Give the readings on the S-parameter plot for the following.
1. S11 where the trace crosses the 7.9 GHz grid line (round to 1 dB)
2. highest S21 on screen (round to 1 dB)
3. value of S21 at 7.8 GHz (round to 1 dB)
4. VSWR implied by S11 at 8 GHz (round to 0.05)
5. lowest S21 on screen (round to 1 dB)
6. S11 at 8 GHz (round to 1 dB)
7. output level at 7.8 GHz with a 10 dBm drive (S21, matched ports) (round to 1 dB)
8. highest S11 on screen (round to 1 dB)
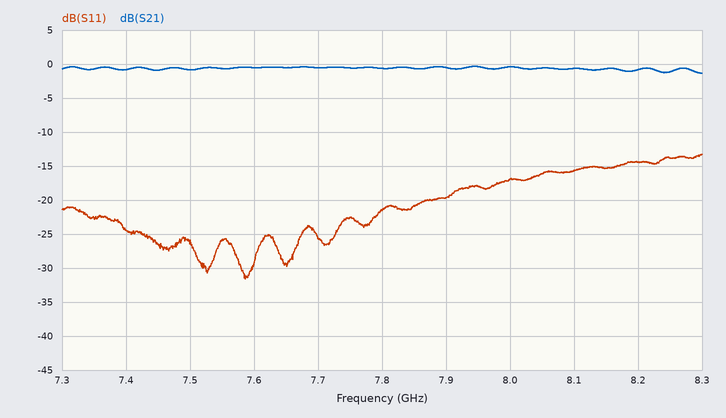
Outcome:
-20 dB
0 dB
-1 dB
1.35
-1 dB
-17 dB
9 dBm
-13 dB
